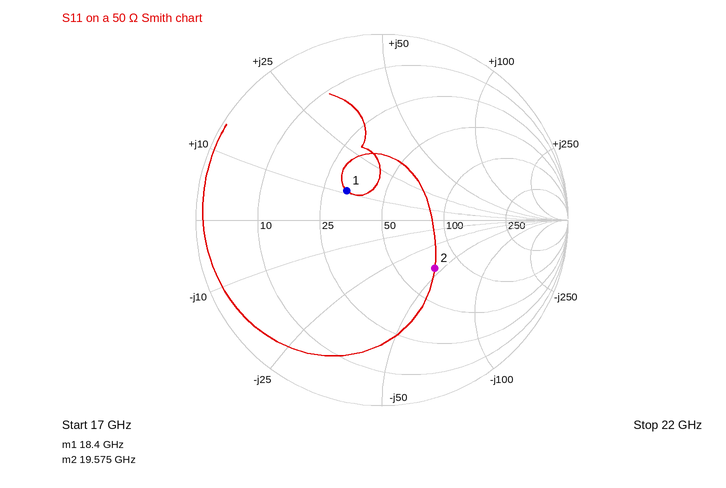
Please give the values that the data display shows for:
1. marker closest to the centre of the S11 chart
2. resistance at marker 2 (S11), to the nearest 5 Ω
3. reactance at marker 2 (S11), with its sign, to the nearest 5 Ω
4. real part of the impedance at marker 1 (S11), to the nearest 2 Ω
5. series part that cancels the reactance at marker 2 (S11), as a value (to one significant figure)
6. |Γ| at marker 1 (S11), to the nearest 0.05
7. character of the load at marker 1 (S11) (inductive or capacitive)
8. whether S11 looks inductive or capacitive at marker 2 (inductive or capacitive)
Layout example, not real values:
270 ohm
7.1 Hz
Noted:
marker 1
75 Ω
-45 Ω
32 Ω
400 pH
0.25
inductive
capacitive
